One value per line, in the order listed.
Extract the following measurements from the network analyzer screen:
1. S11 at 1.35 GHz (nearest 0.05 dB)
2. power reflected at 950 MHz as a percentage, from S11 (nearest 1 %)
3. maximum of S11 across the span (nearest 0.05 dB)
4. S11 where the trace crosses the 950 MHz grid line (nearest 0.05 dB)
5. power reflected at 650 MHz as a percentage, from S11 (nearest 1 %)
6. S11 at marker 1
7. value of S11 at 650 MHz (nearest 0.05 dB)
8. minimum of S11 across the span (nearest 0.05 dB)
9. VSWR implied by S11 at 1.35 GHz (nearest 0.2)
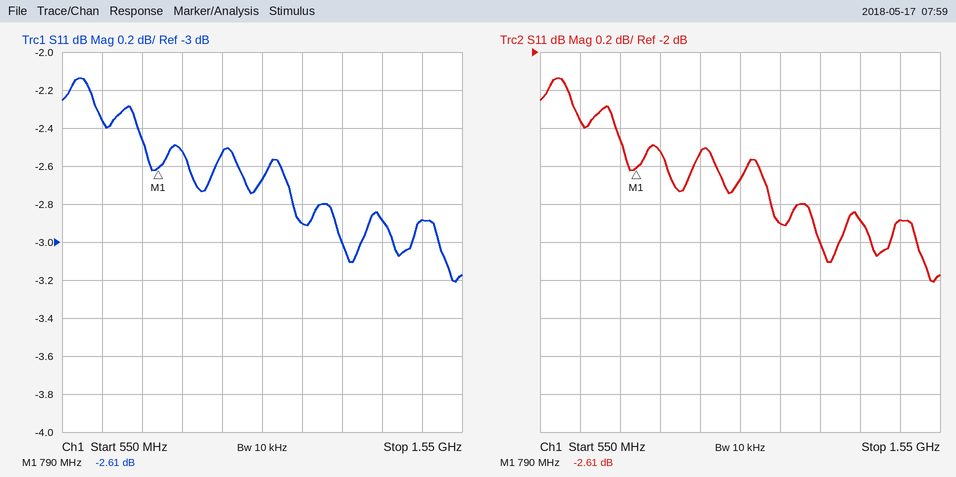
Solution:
-2.90 dB
56 %
-2.15 dB
-2.55 dB
58 %
-2.61 dB
-2.35 dB
-3.20 dB
6.0
